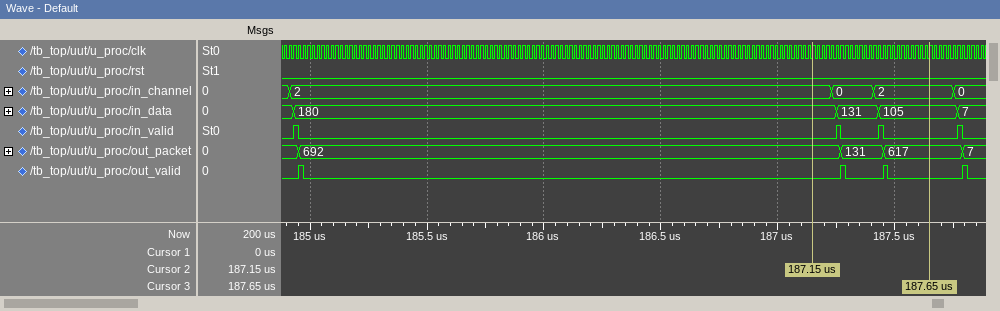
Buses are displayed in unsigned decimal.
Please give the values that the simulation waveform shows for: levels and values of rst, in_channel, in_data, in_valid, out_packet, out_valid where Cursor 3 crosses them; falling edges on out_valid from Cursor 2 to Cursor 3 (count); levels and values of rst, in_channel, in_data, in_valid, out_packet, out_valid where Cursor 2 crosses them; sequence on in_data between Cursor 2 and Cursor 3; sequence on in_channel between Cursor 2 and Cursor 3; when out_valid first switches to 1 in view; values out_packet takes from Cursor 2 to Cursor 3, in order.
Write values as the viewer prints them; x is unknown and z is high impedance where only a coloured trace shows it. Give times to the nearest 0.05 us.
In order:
rst=0, in_channel=2, in_data=105, in_valid=0, out_packet=617, out_valid=0
2
rst=0, in_channel=2, in_data=180, in_valid=0, out_packet=692, out_valid=0
180, 131, 105
2, 0, 2
184.95 us
692, 131, 617
